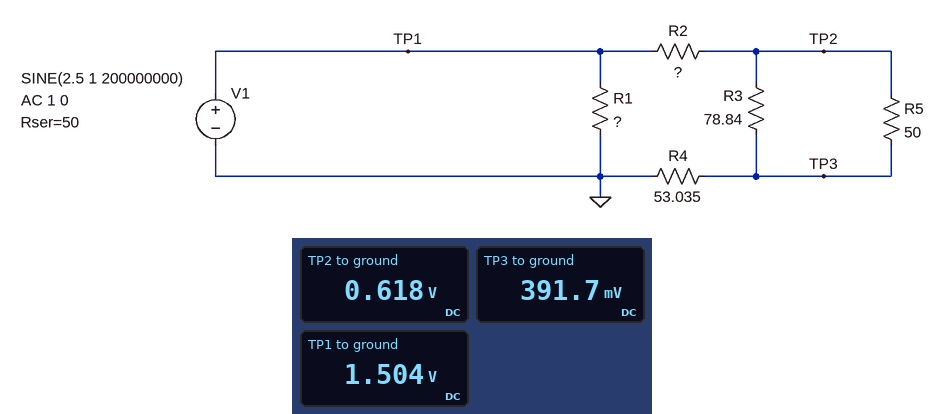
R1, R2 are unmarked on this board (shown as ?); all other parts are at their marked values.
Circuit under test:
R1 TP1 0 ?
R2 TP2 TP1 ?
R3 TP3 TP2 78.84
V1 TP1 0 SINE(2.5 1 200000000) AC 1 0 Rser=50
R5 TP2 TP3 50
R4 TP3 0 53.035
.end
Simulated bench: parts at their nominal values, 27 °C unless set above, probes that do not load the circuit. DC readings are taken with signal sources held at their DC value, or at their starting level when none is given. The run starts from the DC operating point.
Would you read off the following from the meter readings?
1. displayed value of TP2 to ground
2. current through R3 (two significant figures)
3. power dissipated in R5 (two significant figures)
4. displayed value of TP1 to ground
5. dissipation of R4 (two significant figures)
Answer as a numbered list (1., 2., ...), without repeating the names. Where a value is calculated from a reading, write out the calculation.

1. 0.618 V
2. (618 mV - 391.7 mV) / 78.84 Ω = 2.9 mA
3. (618 mV - 391.7 mV)^2 / 50 Ω = 1.0 mW
4. 1.504 V
5. (391.7 mV)^2 / 53.03 Ω = 2.9 mW
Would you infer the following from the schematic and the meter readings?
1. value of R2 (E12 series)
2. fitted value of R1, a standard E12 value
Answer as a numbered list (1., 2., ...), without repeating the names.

1. 120 Ω
2. 120 Ω
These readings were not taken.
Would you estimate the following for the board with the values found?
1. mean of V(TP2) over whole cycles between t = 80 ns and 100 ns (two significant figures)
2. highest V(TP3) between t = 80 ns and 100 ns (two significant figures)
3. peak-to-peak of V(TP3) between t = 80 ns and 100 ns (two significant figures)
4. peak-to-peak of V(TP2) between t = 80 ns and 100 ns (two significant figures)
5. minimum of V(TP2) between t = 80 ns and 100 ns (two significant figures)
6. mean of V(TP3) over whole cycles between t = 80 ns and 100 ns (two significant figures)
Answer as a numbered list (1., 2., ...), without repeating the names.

1. 620 mV
2. 550 mV
3. 310 mV
4. 490 mV
5. 370 mV
6. 390 mV
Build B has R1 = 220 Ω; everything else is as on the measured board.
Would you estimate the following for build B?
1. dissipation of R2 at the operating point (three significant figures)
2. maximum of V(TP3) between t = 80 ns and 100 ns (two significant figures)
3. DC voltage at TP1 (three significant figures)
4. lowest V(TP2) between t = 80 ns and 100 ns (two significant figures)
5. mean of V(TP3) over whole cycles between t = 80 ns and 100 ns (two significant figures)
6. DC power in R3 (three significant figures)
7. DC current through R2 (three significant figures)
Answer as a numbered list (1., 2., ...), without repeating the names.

1. 8.34 mW
2. 620 mV
3. 1.70 V
4. 420 mV
5. 440 mV
6. 825 µW
7. 8.34 mA
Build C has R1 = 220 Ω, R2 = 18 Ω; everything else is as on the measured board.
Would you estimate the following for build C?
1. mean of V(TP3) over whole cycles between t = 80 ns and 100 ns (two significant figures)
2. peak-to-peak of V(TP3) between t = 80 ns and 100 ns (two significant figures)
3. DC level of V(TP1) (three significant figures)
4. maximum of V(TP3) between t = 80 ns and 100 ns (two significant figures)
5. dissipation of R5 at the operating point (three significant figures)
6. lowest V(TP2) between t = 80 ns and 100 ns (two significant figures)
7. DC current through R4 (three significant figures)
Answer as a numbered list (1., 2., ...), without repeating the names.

1. 760 mV
2. 610 mV
3. 1.45 V
4. 1.1 V
5. 3.83 mW
6. 720 mV
7. 14.3 mA
